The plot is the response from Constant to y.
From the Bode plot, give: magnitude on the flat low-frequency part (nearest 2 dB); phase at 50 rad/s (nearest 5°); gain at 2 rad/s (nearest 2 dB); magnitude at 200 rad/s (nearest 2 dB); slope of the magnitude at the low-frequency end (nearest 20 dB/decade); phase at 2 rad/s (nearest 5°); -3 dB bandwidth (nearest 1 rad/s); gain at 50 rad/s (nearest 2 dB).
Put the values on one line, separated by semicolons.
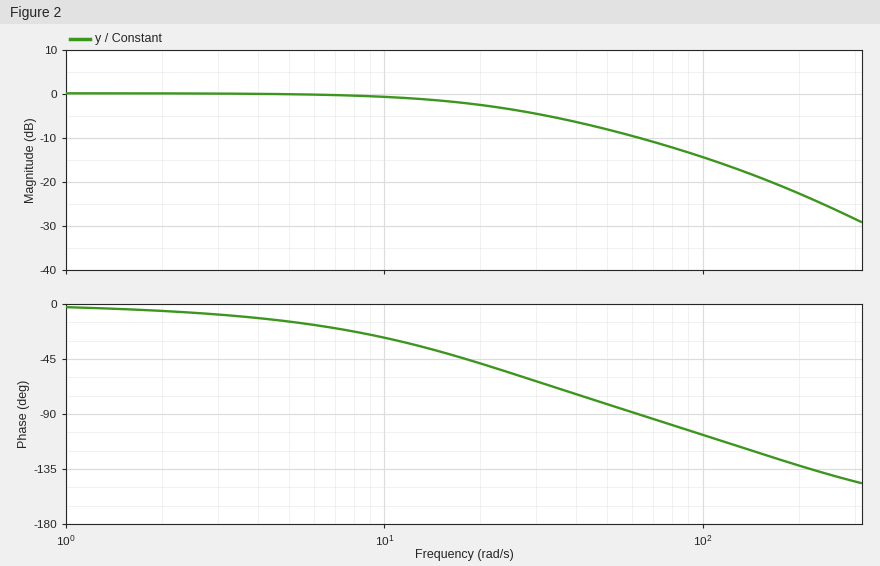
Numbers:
0 dB; -80°; 0 dB; -22 dB; 0 dB/decade; -5°; 22 rad/s; -8 dB
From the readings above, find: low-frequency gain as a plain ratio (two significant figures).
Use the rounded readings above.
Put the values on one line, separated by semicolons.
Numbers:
1.0
